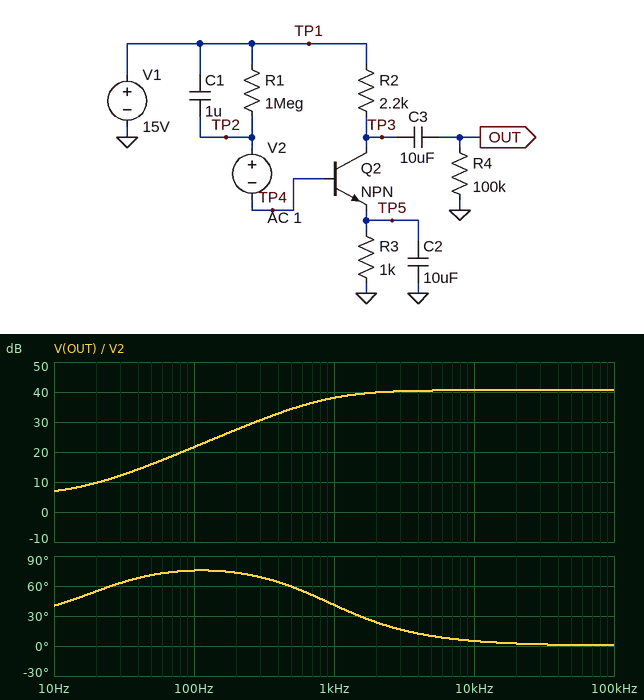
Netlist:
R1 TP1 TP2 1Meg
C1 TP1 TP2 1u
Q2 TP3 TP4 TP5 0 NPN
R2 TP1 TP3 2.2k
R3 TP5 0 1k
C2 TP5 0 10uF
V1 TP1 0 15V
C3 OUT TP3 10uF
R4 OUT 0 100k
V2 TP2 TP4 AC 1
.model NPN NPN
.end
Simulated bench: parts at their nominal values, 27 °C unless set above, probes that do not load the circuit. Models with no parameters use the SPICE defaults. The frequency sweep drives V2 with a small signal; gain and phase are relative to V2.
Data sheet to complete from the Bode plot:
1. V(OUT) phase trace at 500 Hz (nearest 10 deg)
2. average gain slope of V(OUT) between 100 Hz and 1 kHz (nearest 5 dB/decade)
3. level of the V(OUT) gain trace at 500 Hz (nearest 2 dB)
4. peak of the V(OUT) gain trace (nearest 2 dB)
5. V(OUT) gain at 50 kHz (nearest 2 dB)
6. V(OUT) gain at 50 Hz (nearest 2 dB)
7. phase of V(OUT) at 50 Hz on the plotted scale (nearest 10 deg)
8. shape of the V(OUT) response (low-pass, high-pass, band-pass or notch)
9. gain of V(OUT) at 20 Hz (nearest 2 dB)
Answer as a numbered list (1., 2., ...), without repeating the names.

1. 60 deg
2. 15 dB/decade
3. 34 dB
4. 40 dB
5. 40 dB
6. 16 dB
7. 70 deg
8. high-pass
9. 10 dB
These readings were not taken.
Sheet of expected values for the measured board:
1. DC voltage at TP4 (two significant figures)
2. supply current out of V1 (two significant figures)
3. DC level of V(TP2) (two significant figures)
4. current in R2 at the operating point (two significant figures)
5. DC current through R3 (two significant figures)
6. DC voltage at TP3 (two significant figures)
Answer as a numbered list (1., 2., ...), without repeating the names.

1. 2.1 V
2. 1.3 mA
3. 2.1 V
4. 1.3 mA
5. 1.3 mA
6. 12 V
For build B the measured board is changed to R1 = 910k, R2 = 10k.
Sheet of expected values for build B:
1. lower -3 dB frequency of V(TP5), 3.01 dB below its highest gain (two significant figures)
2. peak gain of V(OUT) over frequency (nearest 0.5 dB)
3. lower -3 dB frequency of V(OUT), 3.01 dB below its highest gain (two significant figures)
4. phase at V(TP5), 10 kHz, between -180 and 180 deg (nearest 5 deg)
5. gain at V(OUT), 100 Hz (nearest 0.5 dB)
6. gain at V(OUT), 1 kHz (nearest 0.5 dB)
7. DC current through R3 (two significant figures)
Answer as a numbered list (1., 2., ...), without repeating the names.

1. 12 Hz
2. 50.0 dB
3. 2.1 kHz
4. 100 deg
5. 23.5 dB
6. 42.5 dB
7. 1.4 mA
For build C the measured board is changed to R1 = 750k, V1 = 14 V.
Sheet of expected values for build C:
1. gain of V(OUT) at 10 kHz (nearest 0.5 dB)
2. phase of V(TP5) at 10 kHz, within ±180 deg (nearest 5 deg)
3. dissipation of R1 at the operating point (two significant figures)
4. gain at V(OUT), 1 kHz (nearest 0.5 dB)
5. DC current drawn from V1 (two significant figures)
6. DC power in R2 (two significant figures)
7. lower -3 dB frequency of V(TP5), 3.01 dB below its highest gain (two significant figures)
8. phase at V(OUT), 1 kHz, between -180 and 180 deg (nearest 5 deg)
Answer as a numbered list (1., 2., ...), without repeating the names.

1. 42.0 dB
2. 95 deg
3. 180 µW
4. 39.0 dB
5. 1.6 mA
6. 5.3 mW
7. 1.6 Hz
8. 45 deg
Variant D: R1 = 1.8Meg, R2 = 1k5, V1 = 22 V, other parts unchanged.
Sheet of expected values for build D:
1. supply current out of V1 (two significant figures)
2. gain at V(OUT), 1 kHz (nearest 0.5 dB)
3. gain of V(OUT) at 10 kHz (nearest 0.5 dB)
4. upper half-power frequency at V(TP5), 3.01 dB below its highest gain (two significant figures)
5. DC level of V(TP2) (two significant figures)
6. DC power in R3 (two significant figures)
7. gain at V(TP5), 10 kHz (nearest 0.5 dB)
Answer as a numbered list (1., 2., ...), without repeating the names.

1. 1.1 mA
2. 34.0 dB
3. 36.0 dB
4. 780 Hz
5. 1.9 V
6. 1.3 mW
7. -23.0 dB
